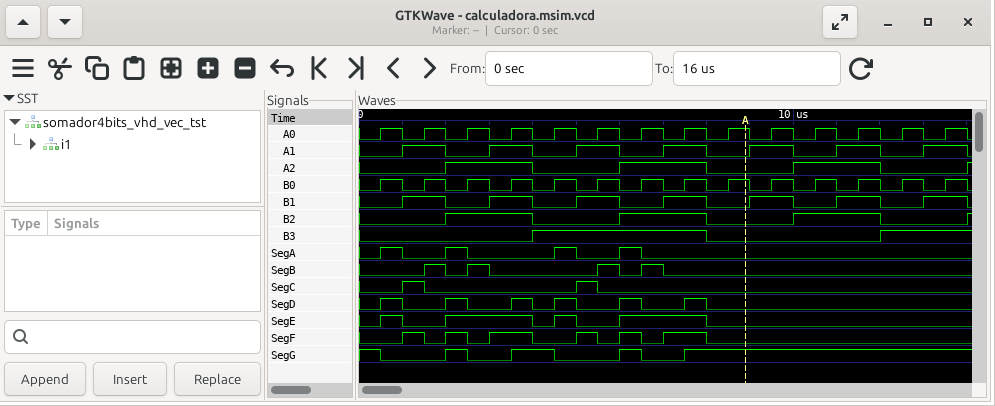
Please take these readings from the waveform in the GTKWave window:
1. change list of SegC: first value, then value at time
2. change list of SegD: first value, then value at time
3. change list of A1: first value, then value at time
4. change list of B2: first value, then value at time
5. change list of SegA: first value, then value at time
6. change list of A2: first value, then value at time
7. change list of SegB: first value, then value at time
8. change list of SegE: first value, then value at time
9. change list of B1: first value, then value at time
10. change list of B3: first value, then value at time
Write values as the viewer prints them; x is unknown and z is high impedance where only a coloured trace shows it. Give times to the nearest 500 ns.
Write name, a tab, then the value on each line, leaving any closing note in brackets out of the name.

change list of SegC: first value, then value at time	0, 1 at 1000 ns, 0 at 1500 ns, 1 at 5000 ns, 0 at 5500 ns
change list of SegD: first value, then value at time	0, 1 at 500 ns, 0 at 1000 ns, 1 at 2000 ns, 0 at 2500 ns, 1 at 3500 ns, 0 at 4000 ns, 1 at 4500 ns, 0 at 5000 ns, 1 at 6000 ns, 0 at 6500 ns, 1 at 7500 ns, 0 at 8000 ns
change list of A1: first value, then value at time	0, 1 at 1000 ns, 0 at 2000 ns, 1 at 3000 ns, 0 at 4000 ns, 1 at 5000 ns, 0 at 6000 ns, 1 at 7000 ns, 0 at 8000 ns, 1 at 9000 ns, 0 at 10000 ns, 1 at 11000 ns, 0 at 12000 ns, 1 at 13000 ns, 0 at 14000 ns
change list of B2: first value, then value at time	0, 1 at 2000 ns, 0 at 4000 ns, 1 at 6000 ns, 0 at 8000 ns, 1 at 10000 ns, 0 at 12000 ns, 1 at 14000 ns
change list of SegA: first value, then value at time	0, 1 at 500 ns, 0 at 1000 ns, 1 at 2000 ns, 0 at 2500 ns, 1 at 4500 ns, 0 at 5000 ns, 1 at 6000 ns, 0 at 6500 ns
change list of A2: first value, then value at time	0, 1 at 2000 ns, 0 at 4000 ns, 1 at 6000 ns, 0 at 8000 ns, 1 at 10000 ns, 0 at 12000 ns, 1 at 14000 ns
change list of SegB: first value, then value at time	0, 1 at 1500 ns, 0 at 2000 ns, 1 at 2500 ns, 0 at 3000 ns, 1 at 5500 ns, 0 at 6000 ns, 1 at 6500 ns, 0 at 7000 ns
change list of SegE: first value, then value at time	0, 1 at 500 ns, 0 at 1000 ns, 1 at 2000 ns, 0 at 4000 ns, 1 at 4500 ns, 0 at 5000 ns, 1 at 6000 ns, 0 at 8000 ns
change list of B1: first value, then value at time	0, 1 at 1000 ns, 0 at 2000 ns, 1 at 3000 ns, 0 at 4000 ns, 1 at 5000 ns, 0 at 6000 ns, 1 at 7000 ns, 0 at 8000 ns, 1 at 9000 ns, 0 at 10000 ns, 1 at 11000 ns, 0 at 12000 ns, 1 at 13000 ns, 0 at 14000 ns
change list of B3: first value, then value at time	0, 1 at 4000 ns, 0 at 8000 ns, 1 at 12000 ns
